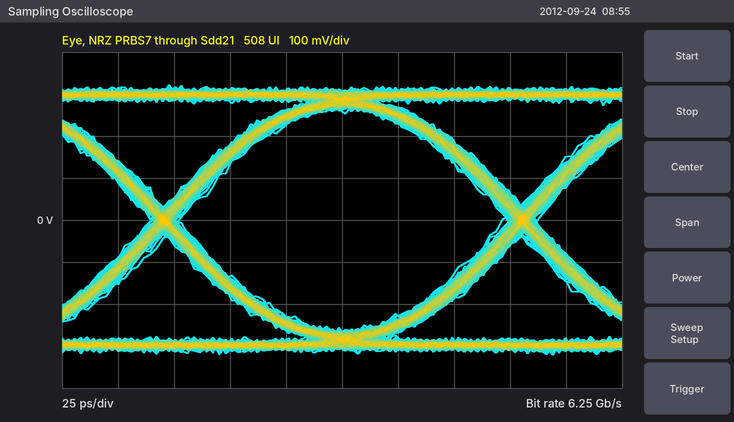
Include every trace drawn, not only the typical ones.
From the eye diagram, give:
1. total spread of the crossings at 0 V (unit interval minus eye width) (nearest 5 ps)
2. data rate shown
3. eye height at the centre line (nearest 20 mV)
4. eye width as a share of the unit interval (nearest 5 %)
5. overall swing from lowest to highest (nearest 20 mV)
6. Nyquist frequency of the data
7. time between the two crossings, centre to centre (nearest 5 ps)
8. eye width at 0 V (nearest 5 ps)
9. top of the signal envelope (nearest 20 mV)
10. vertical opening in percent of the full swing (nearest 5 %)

15 ps
6.25 Gb/s
520 mV
90 %
640 mV
3.125 GHz
160 ps
145 ps
320 mV
80 %
